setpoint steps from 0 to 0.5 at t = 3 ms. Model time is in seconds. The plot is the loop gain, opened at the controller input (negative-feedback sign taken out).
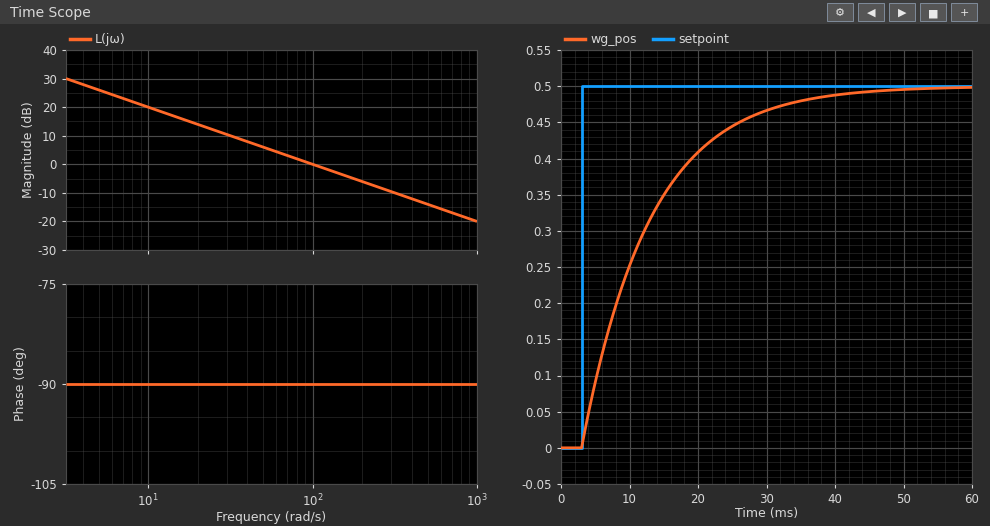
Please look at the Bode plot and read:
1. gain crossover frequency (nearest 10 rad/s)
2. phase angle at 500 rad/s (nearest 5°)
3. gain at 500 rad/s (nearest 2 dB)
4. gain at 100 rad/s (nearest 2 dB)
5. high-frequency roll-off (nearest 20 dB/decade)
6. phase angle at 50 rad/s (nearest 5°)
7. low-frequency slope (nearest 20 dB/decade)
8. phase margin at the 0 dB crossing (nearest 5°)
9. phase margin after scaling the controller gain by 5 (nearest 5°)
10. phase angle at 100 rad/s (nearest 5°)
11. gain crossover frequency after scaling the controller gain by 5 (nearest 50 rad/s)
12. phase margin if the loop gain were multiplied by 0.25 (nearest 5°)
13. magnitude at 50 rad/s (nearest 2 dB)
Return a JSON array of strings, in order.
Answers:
["100 rad/s", "-90°", "-14 dB", "0 dB", "-20 dB/decade", "-90°", "-20 dB/decade", "90°", "90°", "-90°", "500 rad/s", "90°", "6 dB"]
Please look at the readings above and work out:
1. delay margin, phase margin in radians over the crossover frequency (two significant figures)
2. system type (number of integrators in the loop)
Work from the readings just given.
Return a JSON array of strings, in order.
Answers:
["0.016 s", "1"]
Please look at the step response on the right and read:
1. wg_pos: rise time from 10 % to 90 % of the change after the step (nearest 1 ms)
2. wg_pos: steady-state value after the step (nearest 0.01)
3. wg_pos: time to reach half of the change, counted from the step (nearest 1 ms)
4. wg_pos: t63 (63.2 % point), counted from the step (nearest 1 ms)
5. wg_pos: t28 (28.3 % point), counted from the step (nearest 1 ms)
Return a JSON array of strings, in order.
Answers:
["22 ms", "0.50", "7 ms", "10 ms", "3 ms"]
